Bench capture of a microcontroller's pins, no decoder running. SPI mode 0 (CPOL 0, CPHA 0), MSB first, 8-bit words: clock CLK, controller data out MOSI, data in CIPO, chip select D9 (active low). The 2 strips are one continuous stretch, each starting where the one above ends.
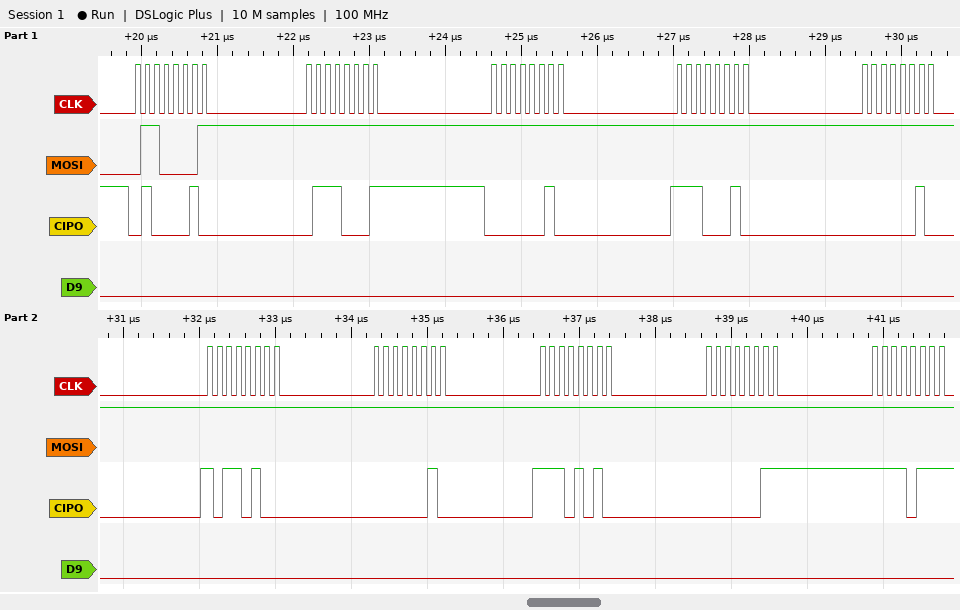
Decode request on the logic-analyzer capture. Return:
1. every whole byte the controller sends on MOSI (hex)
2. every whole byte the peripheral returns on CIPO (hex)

61 FF FF FF FF FF FF FF FF FF
42 71 02 E2 02 B4 02 EA 03 F7
